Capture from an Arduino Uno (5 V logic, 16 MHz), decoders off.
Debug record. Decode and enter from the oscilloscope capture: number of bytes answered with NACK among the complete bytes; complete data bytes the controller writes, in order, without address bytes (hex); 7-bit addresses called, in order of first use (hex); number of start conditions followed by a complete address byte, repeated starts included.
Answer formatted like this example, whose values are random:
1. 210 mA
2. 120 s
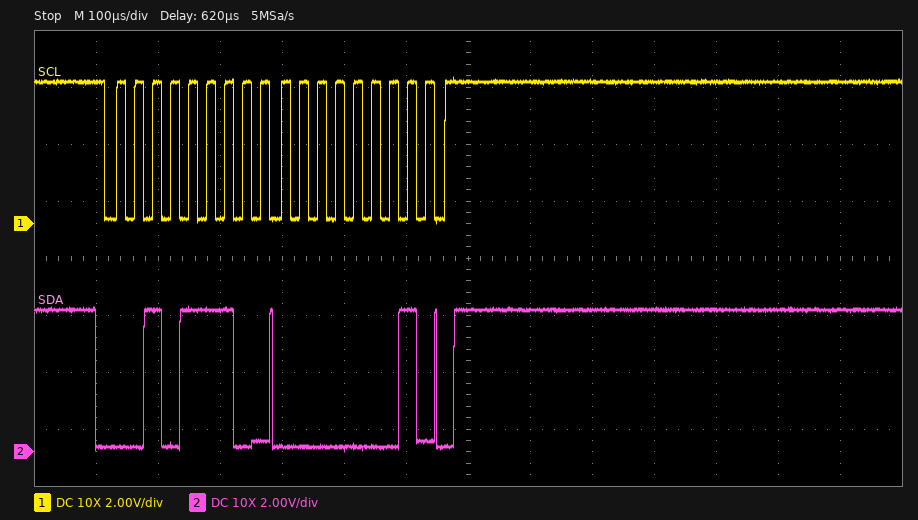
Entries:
1. 0
2. 01
3. 0x17
4. 1
